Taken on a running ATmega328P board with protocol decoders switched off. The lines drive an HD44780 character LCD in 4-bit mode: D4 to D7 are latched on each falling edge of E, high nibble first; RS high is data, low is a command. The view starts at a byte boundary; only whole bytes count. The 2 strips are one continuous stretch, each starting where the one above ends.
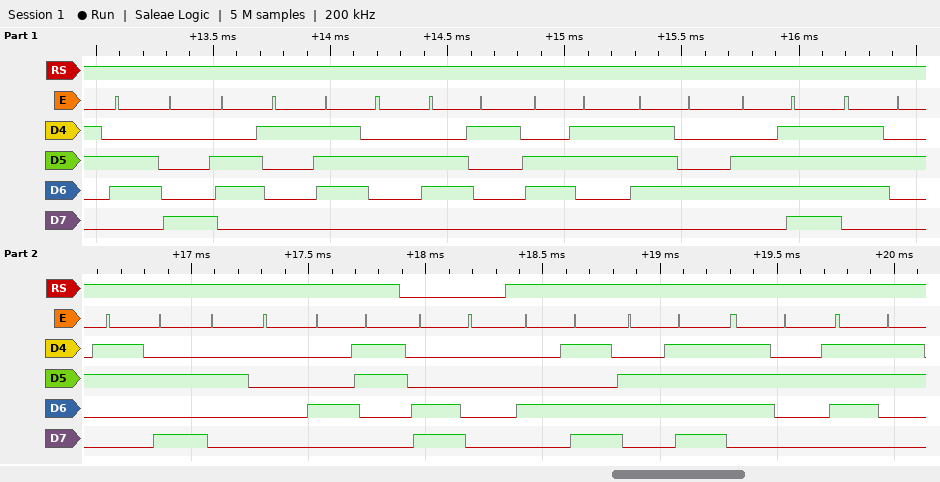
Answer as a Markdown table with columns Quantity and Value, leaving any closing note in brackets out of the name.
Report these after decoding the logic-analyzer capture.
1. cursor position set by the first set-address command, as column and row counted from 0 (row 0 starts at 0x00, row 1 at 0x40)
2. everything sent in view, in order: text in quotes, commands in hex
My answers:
| Quantity | Value |
|---|---|
| cursor position set by the first set-address command, as column and row counted from 0 | column 0, row 1 |
| everything sent in view, in order: text in quotes, commands in hex | "haractor: C" 0xC0 "Mors" |
